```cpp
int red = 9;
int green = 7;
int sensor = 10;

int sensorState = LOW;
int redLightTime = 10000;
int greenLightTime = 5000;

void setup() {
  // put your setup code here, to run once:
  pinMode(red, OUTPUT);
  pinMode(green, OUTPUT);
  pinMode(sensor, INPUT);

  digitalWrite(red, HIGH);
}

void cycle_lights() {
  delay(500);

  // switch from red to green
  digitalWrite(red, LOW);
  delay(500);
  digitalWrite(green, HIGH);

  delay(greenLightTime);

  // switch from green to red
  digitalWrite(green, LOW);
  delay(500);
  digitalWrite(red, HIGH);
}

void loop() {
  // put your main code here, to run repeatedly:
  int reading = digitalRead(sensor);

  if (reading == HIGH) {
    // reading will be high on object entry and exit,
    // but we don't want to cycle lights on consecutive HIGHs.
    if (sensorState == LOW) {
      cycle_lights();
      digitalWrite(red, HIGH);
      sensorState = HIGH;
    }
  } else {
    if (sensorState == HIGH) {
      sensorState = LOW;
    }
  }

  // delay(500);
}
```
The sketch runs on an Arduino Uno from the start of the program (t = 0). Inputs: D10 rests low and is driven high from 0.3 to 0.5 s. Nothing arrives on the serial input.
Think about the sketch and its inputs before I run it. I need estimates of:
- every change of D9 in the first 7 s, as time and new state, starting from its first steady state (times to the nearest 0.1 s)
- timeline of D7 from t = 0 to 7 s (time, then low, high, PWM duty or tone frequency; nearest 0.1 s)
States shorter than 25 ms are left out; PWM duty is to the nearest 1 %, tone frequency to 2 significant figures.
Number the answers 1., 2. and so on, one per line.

1. 0 s high; 0.8 s low; 6.8 s high
2. 0 s low; 1.3 s high; 6.3 s low
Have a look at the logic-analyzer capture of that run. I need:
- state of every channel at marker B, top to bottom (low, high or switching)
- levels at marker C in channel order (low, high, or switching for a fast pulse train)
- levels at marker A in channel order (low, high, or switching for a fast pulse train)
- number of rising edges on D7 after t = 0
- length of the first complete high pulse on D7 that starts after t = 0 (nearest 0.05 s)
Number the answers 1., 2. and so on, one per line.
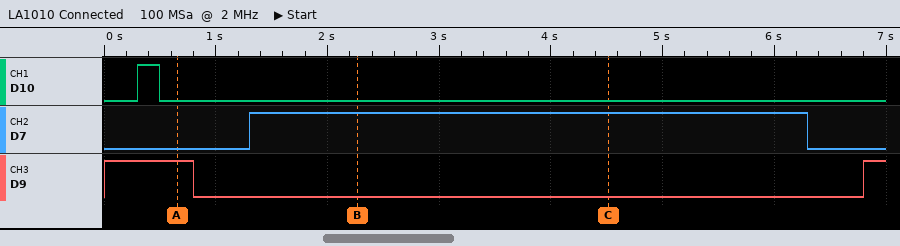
1. D10 low, D7 high, D9 low
2. D10 low, D7 high, D9 low
3. D10 low, D7 low, D9 high
4. 1
5. 5.00 s
